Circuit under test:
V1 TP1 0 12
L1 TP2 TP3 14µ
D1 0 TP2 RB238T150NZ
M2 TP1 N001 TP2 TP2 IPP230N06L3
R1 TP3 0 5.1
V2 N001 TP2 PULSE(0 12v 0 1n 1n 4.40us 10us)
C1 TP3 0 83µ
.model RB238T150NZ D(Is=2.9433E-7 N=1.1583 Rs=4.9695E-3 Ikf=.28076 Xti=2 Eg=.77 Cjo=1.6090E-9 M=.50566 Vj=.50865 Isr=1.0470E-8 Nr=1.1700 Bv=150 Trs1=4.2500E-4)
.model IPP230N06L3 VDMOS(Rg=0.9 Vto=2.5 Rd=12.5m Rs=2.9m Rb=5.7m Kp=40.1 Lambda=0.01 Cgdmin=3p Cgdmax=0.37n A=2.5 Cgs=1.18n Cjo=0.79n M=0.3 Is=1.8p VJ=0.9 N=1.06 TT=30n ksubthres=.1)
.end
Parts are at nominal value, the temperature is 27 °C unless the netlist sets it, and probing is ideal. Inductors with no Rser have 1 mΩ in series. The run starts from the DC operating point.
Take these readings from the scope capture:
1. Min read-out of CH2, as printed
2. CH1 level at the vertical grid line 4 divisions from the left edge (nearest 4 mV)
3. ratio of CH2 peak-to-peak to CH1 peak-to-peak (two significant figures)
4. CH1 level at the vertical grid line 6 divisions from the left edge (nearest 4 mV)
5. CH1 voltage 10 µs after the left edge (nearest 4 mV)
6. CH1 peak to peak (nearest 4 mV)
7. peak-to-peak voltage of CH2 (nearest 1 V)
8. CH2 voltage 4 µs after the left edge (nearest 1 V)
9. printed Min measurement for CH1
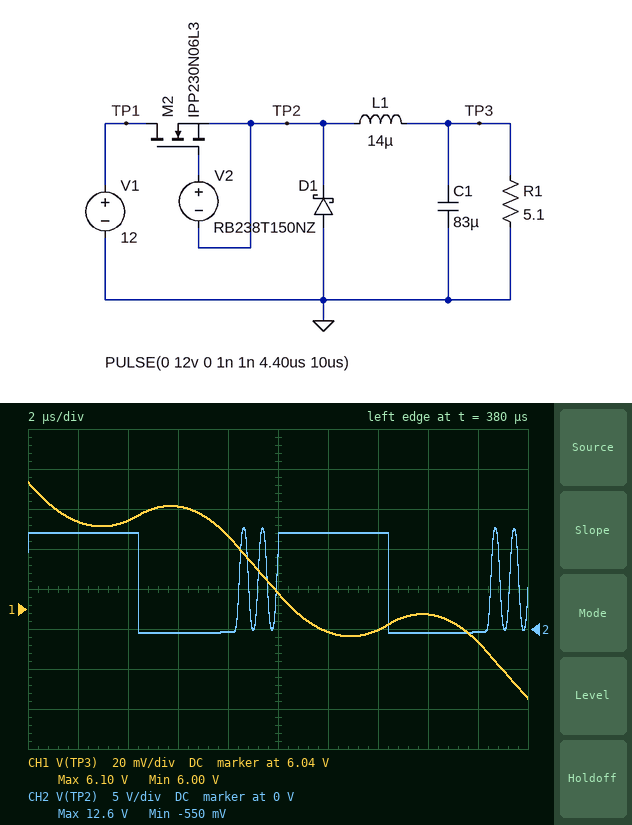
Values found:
-550 mV
6.076 V
120
6.028 V
6.048 V
108 mV
13 V
12 V
6.00 V
